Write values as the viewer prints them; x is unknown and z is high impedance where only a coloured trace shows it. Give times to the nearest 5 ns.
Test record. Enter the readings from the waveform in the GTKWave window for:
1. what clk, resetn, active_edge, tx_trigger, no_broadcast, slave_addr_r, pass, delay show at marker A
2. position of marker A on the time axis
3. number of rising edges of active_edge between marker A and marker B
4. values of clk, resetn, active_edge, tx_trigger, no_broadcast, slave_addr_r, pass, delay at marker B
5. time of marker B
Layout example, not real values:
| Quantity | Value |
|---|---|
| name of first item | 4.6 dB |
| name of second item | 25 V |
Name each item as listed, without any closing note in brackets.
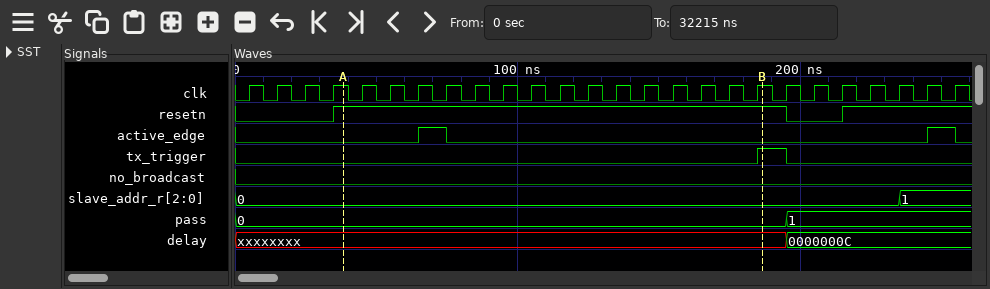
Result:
| Quantity | Value |
|---|---|
| what clk, resetn, active_edge, tx_trigger, no_broadcast, slave_addr_r, pass, delay show at marker A | clk=1, resetn=1, active_edge=0, tx_trigger=0, no_broadcast=0, slave_addr_r=0, pass=0, delay=xxxxxxxx |
| position of marker A on the time axis | 40 ns |
| number of rising edges of active_edge between marker A and marker B | 1 |
| values of clk, resetn, active_edge, tx_trigger, no_broadcast, slave_addr_r, pass, delay at marker B | clk=1, resetn=1, active_edge=0, tx_trigger=1, no_broadcast=0, slave_addr_r=0, pass=0, delay=xxxxxxxx |
| time of marker B | 185 ns |
